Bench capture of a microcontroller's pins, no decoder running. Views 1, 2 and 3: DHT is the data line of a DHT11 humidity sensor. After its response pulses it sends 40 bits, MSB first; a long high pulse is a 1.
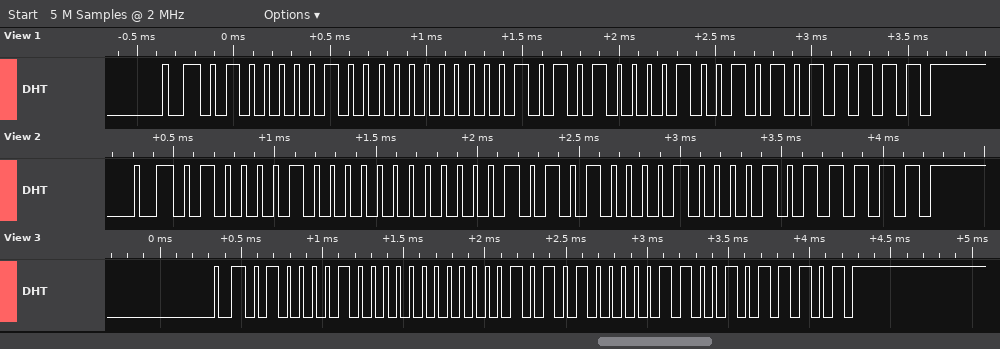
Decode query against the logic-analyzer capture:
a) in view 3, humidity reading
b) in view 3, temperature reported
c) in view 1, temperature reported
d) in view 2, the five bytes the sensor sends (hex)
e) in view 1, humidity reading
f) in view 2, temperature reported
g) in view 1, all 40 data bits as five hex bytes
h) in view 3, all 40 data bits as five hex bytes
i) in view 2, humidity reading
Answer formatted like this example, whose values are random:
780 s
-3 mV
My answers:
66 %
21.6 °C
21.9 °C
42 00 15 08 5F
65 %
21.8 °C
41 00 15 09 5F
42 00 15 06 5D
66 %
